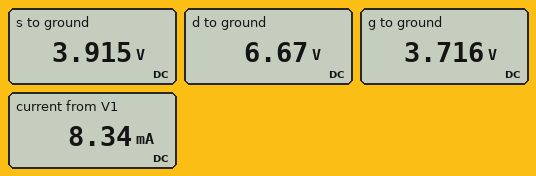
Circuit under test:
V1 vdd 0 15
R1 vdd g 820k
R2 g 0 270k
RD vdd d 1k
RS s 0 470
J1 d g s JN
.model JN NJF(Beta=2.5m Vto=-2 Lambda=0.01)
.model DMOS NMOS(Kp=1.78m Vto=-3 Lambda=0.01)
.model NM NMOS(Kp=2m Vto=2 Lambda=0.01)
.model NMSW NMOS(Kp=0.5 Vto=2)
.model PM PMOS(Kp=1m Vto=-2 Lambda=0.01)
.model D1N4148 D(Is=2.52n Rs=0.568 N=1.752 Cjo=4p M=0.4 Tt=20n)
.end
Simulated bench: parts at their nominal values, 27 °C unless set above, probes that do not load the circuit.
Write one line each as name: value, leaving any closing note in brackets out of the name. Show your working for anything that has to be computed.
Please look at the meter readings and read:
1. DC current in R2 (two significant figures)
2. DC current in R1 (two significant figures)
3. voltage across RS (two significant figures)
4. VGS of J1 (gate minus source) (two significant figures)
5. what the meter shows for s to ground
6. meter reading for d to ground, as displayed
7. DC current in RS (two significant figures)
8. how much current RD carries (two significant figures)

DC current in R2: (3.716 V) / 270 kΩ = 14 µA
DC current in R1: (15 V - 3.716 V) / 820 kΩ = 14 µA
voltage across RS: 3.915 V = 3.9 V
VGS of J1 (gate minus source): 3.716 V - 3.915 V = -200 mV
what the meter shows for s to ground: 3.915 V
meter reading for d to ground, as displayed: 6.67 V
DC current in RS: (3.915 V) / 470 Ω = 8.3 mA
how much current RD carries: (15 V - 6.67 V) / 1 kΩ = 8.3 mA
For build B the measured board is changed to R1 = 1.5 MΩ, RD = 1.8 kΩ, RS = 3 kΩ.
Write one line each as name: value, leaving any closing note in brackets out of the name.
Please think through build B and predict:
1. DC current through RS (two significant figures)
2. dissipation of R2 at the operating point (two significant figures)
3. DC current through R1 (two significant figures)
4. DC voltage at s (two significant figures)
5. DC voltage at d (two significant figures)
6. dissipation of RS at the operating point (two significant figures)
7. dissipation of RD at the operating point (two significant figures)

DC current through RS: 1.2 mA
dissipation of R2 at the operating point: 19 µW
DC current through R1: 8.5 µA
DC voltage at s: 3.6 V
DC voltage at d: 13 V
dissipation of RS at the operating point: 4.4 mW
dissipation of RD at the operating point: 2.6 mW
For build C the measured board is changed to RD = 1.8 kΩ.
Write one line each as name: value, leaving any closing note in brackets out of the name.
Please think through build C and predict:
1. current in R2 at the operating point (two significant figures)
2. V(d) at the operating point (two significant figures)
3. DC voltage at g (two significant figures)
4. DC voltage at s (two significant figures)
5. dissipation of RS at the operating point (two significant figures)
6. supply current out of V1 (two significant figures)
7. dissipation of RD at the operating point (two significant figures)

current in R2 at the operating point: 13 µA
V(d) at the operating point: 3.6 V
DC voltage at g: 3.5 V
DC voltage at s: 3.0 V
dissipation of RS at the operating point: 19 mW
supply current out of V1: 6.4 mA
dissipation of RD at the operating point: 73 mW
